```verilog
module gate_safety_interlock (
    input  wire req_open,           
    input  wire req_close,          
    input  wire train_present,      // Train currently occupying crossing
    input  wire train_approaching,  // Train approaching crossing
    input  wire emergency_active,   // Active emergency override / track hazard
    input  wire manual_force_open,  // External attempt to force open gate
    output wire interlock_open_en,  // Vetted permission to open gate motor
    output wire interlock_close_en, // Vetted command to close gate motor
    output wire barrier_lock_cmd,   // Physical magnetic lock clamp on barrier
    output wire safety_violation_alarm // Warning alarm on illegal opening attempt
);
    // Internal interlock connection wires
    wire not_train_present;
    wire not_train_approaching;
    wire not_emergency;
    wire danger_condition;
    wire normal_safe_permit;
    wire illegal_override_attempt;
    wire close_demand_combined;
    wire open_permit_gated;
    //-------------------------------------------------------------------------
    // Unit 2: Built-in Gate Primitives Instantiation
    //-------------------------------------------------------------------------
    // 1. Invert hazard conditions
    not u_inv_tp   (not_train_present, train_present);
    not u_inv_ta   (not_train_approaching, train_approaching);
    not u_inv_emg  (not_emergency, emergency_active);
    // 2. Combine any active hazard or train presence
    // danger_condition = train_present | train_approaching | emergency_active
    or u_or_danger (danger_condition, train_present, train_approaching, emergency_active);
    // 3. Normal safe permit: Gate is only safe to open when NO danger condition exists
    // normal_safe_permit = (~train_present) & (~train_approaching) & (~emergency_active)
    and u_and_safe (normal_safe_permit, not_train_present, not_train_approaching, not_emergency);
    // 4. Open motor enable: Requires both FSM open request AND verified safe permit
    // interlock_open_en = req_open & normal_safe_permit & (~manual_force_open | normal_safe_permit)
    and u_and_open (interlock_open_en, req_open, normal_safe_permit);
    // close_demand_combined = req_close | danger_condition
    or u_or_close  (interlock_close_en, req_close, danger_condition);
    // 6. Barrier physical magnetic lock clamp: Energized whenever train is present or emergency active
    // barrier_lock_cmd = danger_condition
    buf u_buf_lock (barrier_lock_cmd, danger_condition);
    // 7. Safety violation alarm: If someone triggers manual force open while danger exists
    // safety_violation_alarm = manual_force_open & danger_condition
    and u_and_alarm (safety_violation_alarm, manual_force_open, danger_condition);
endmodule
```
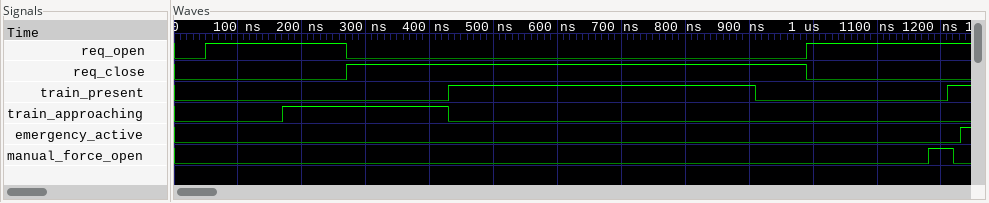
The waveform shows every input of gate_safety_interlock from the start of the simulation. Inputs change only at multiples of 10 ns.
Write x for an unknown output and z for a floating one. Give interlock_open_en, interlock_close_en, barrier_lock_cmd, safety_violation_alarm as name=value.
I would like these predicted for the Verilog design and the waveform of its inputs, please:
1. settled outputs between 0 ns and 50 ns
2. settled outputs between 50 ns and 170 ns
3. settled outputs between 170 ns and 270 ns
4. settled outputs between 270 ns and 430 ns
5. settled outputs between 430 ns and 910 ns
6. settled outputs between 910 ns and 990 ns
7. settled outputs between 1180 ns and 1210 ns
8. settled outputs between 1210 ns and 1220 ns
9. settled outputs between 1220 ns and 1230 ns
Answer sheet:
interlock_open_en=0, interlock_close_en=0, barrier_lock_cmd=0, safety_violation_alarm=0
interlock_open_en=1, interlock_close_en=0, barrier_lock_cmd=0, safety_violation_alarm=0
interlock_open_en=0, interlock_close_en=1, barrier_lock_cmd=1, safety_violation_alarm=0
interlock_open_en=0, interlock_close_en=1, barrier_lock_cmd=1, safety_violation_alarm=0
interlock_open_en=0, interlock_close_en=1, barrier_lock_cmd=1, safety_violation_alarm=0
interlock_open_en=0, interlock_close_en=1, barrier_lock_cmd=0, safety_violation_alarm=0
interlock_open_en=1, interlock_close_en=0, barrier_lock_cmd=0, safety_violation_alarm=0
interlock_open_en=0, interlock_close_en=1, barrier_lock_cmd=1, safety_violation_alarm=1
interlock_open_en=0, interlock_close_en=1, barrier_lock_cmd=1, safety_violation_alarm=0
